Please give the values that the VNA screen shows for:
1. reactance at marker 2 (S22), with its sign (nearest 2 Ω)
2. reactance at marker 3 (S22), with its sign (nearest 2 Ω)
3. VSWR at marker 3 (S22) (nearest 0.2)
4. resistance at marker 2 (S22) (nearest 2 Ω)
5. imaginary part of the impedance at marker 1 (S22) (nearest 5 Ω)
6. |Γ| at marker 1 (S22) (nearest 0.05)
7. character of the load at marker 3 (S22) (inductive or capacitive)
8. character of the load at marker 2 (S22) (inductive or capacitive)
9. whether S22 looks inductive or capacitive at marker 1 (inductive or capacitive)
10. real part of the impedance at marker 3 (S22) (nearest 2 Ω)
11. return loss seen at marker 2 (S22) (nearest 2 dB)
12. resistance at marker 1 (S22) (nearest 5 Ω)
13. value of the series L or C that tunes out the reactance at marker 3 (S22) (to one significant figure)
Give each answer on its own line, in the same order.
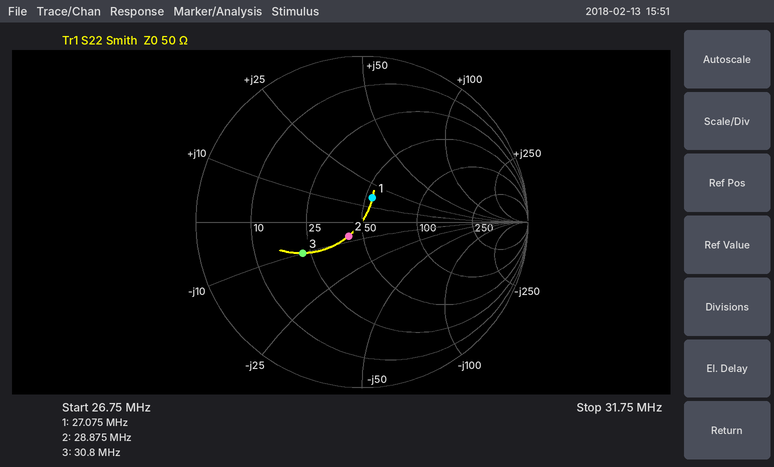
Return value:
-8 Ω
-10 Ω
2.4
42 Ω
+15 Ω
0.15
capacitive
capacitive
inductive
22 Ω
18 dB
55 Ω
50 nH
